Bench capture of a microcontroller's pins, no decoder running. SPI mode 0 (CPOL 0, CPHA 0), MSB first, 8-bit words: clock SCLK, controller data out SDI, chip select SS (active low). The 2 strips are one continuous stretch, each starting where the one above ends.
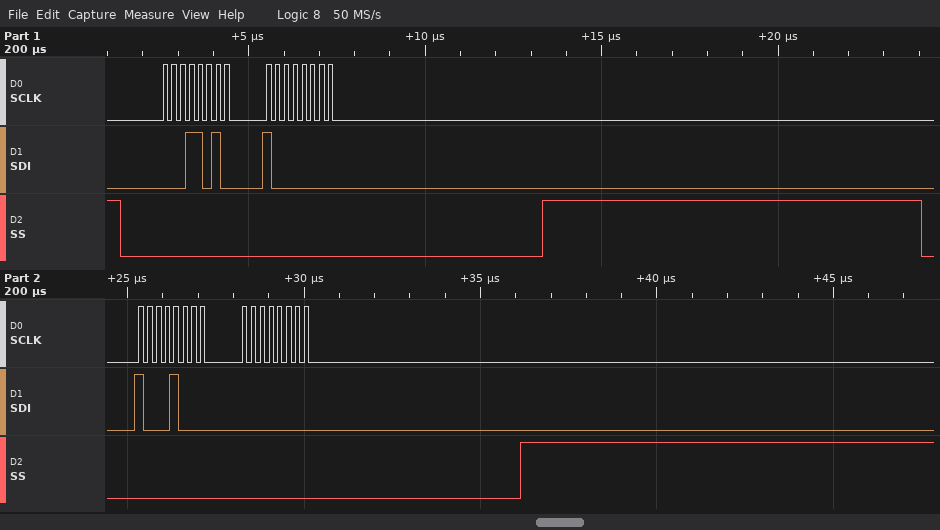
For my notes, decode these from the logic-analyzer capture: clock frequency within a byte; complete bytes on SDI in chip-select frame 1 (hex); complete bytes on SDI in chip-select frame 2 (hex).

4 MHz
0x1A 0x80
0x88 0x00
